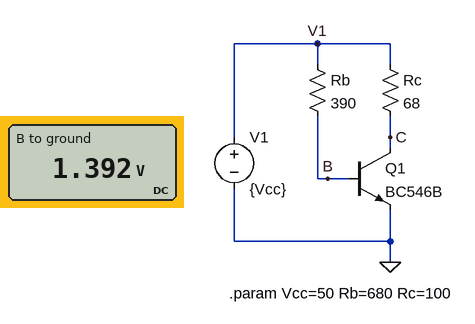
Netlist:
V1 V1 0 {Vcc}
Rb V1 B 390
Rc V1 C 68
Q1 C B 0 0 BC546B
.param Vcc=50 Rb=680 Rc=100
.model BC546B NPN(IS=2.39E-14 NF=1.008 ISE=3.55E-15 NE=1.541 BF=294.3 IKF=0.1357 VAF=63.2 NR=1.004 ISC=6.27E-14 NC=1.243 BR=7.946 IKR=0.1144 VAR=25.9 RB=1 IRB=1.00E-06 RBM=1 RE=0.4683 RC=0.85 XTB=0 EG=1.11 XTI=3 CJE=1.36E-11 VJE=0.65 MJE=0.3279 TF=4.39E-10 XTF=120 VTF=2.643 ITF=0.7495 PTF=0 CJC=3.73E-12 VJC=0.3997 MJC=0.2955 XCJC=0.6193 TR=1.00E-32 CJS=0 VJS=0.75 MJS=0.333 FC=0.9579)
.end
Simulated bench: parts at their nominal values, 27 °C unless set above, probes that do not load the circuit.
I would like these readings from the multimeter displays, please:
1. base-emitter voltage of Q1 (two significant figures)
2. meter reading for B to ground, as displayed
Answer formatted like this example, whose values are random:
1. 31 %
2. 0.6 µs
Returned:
1. 1.4 V
2. 1.392 V
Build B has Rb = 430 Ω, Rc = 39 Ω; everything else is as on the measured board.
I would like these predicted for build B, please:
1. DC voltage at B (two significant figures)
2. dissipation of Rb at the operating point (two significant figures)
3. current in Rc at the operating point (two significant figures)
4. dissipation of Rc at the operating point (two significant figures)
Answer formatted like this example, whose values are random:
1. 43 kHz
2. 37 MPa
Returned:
1. 1.6 V
2. 5.4 W
3. 1.2 A
4. 60 W
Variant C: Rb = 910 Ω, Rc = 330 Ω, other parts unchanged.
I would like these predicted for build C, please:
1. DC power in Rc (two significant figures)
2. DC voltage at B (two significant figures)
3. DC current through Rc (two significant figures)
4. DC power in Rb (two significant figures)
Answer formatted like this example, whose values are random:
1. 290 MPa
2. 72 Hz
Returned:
1. 7.5 W
2. 970 mV
3. 150 mA
4. 2.6 W
